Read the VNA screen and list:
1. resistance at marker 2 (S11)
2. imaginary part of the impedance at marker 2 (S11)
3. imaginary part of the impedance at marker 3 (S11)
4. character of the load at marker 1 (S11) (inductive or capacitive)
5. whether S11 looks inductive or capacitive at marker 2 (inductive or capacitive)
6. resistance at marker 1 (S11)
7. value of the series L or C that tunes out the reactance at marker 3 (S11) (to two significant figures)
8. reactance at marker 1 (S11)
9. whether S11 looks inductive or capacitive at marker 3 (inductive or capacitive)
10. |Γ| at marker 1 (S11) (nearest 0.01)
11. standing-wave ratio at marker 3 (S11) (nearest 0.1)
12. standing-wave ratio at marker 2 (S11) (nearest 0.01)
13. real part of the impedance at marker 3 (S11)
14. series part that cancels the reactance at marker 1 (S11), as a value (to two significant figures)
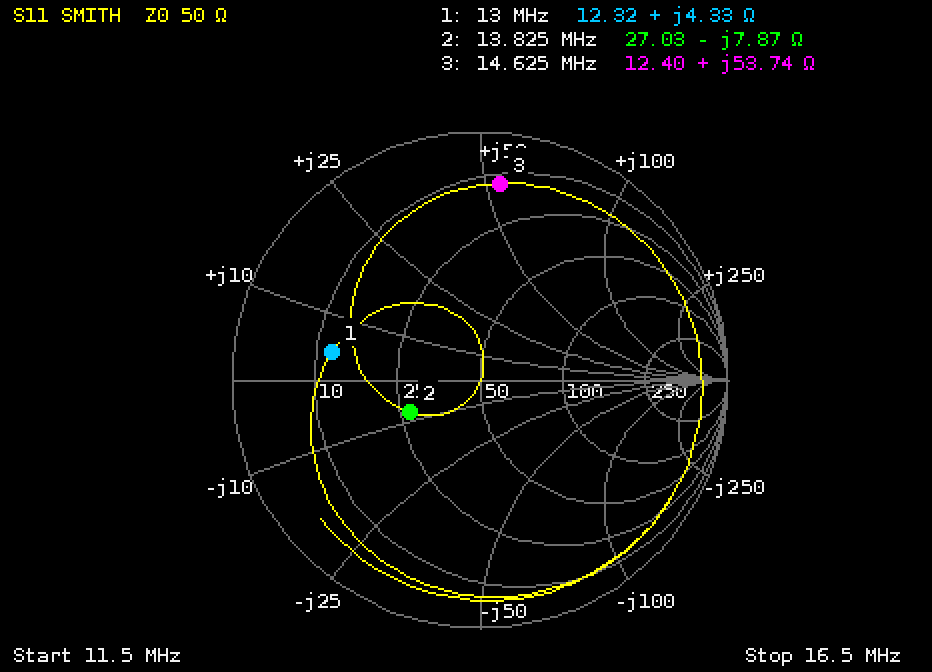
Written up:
27.03 Ω
-7.87 Ω
+53.74 Ω
inductive
capacitive
12.32 Ω
200 pF
+4.33 Ω
inductive
0.61
8.8
1.91
12.40 Ω
2.8 nF
